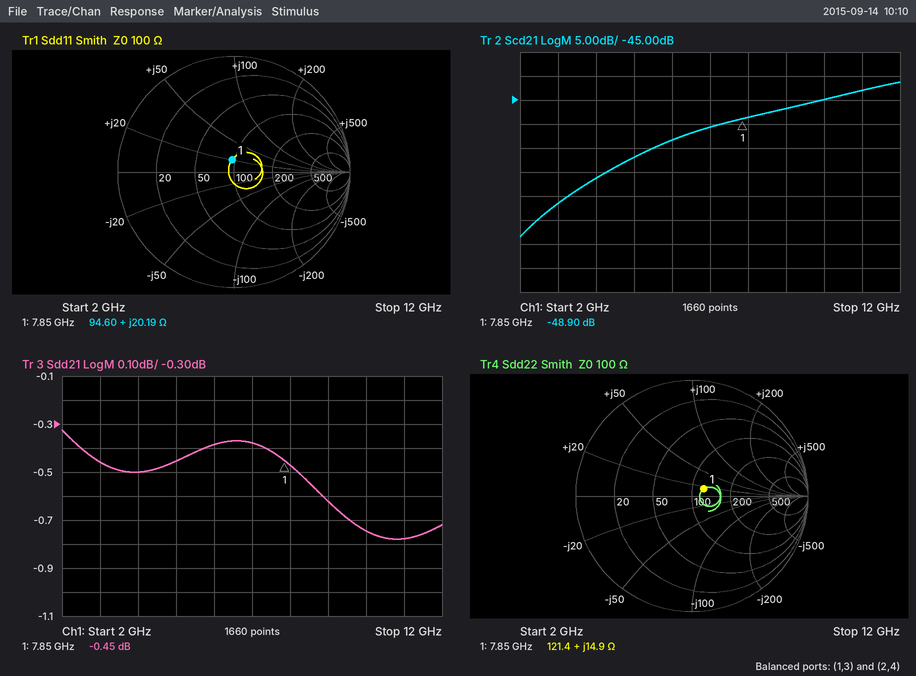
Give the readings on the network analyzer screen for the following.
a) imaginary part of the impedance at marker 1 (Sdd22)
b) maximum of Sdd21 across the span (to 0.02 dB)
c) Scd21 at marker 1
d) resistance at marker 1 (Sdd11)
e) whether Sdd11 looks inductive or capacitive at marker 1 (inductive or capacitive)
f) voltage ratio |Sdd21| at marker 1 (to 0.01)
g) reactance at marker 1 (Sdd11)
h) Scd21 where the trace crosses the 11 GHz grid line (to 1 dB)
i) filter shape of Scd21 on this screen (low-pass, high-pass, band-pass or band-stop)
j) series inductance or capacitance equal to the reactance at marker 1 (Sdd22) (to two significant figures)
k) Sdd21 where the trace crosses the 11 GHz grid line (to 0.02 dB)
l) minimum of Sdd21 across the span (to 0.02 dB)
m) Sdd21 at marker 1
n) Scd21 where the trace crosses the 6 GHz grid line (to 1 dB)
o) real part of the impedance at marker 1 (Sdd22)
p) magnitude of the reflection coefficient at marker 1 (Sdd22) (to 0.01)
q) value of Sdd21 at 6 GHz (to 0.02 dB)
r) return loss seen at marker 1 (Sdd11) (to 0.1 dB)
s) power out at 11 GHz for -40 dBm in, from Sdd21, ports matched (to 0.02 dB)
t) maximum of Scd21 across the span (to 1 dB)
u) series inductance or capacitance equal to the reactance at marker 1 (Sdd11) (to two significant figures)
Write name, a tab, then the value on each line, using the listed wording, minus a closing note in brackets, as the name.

imaginary part of the impedance at marker 1	+14.9 Ω
maximum of Sdd21 across the span	-0.32 dB
Scd21 at marker 1	-48.90 dB
resistance at marker 1	94.60 Ω
whether Sdd11 looks inductive or capacitive at marker 1	inductive
voltage ratio |Sdd21| at marker 1	0.95
reactance at marker 1	+20.19 Ω
Scd21 where the trace crosses the 11 GHz grid line	-43 dB
filter shape of Scd21 on this screen	high-pass
series inductance or capacitance equal to the reactance at marker 1 (Sdd22)	300 pH
Sdd21 where the trace crosses the 11 GHz grid line	-0.78 dB
minimum of Sdd21 across the span	-0.78 dB
Sdd21 at marker 1	-0.45 dB
Scd21 where the trace crosses the 6 GHz grid line	-53 dB
real part of the impedance at marker 1	121.4 Ω
magnitude of the reflection coefficient at marker 1 (Sdd22)	0.12
value of Sdd21 at 6 GHz	-0.38 dB
return loss seen at marker 1 (Sdd11)	19.4 dB
power out at 11 GHz for -40 dBm in, from Sdd21, ports matched	-40.78 dBm
maximum of Scd21 across the span	-41 dB
series inductance or capacitance equal to the reactance at marker 1 (Sdd11)	410 pH
